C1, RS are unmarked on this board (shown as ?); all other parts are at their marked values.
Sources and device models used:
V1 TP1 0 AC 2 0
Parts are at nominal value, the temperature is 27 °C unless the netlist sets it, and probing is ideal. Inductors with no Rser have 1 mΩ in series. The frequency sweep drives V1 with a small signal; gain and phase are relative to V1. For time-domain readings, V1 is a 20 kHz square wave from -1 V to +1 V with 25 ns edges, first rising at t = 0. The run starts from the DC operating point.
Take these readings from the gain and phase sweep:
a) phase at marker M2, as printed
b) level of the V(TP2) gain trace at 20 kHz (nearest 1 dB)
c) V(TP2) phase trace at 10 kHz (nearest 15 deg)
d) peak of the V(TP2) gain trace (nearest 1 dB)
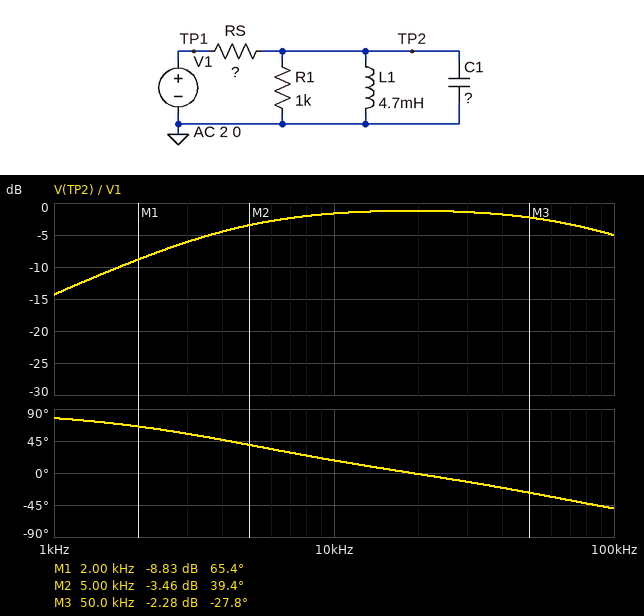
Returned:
39.4 deg
-1 dB
15 deg
-1 dB
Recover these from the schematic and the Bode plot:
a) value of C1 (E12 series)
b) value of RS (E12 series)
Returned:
15 nF
150 Ω
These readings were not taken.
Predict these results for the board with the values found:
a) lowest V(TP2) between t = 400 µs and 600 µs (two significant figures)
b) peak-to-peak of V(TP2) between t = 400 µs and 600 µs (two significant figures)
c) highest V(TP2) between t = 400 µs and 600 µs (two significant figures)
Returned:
-1.0 V
2.0 V
1.0 V
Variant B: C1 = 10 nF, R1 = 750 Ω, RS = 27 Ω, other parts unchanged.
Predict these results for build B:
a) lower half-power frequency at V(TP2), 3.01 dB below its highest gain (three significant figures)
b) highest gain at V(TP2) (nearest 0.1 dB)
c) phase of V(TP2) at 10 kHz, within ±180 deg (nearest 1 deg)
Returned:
881 Hz
-0.3 dB
4 deg
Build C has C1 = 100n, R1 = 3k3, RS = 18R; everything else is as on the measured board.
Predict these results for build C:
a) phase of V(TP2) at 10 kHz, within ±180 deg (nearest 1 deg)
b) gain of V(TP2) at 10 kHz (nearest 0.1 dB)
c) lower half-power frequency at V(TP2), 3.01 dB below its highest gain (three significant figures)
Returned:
-3 deg
-0.1 dB
602 Hz
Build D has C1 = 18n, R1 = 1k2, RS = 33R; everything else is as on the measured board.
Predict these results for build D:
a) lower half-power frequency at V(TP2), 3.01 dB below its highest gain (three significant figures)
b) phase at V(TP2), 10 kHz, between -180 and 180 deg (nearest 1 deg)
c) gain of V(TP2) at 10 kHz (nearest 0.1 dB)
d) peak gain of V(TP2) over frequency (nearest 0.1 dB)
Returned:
1.08 kHz
4 deg
-0.3 dB
-0.2 dB
